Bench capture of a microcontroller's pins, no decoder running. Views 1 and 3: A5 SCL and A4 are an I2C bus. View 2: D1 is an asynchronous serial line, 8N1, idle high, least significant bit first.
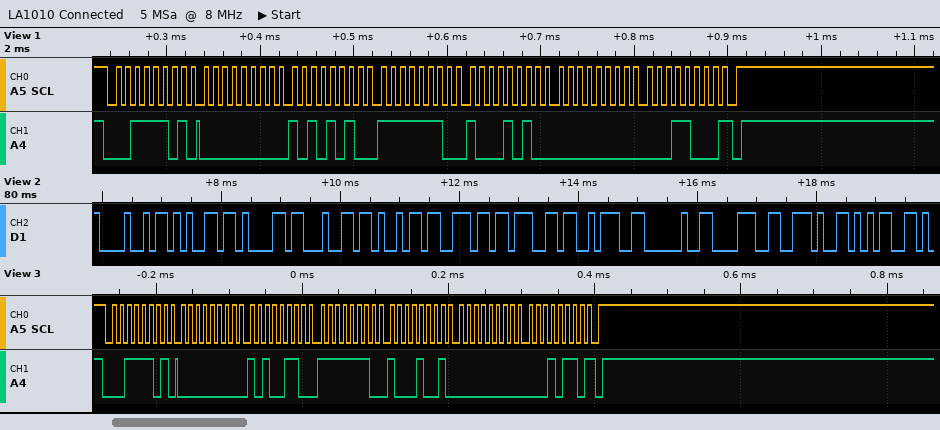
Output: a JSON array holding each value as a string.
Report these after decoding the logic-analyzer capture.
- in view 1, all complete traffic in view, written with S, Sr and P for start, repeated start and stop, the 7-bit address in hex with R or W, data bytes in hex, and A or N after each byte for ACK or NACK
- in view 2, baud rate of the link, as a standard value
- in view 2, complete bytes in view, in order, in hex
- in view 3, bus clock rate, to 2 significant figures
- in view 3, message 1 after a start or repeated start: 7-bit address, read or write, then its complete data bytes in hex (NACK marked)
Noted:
["S 1ER A 00 A AA A FE A 8A A 00 A 18 N P", "9600 baud", "48 65 61 64 69 6E 67 3A 20 38 2E 35", "100 kHz", "0x1E read: 00 A6 FE 89 00 16 NACK"]
